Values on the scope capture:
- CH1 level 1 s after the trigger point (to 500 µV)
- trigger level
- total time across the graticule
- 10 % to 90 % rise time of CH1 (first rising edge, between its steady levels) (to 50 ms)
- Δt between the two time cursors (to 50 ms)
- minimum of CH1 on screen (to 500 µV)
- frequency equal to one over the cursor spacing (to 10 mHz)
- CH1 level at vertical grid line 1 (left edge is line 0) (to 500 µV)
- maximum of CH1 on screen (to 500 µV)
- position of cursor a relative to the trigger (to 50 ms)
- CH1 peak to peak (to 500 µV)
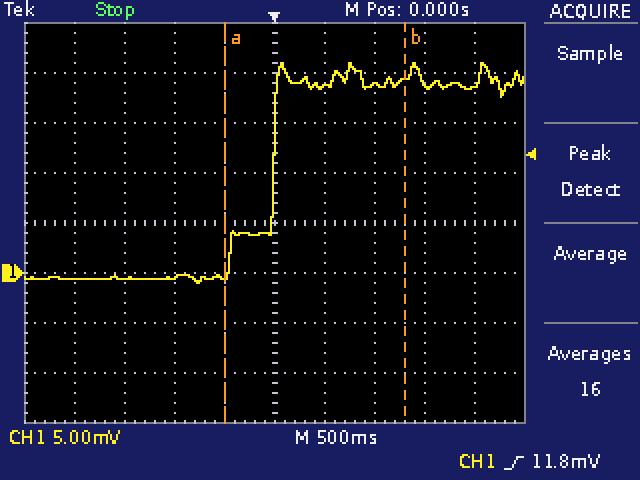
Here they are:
19.0 mV
11.8 mV
5 s
450 ms
1.80 s
-1.0 mV
560 mHz
-500 µV
21.0 mV
-500 ms
22.0 mV
